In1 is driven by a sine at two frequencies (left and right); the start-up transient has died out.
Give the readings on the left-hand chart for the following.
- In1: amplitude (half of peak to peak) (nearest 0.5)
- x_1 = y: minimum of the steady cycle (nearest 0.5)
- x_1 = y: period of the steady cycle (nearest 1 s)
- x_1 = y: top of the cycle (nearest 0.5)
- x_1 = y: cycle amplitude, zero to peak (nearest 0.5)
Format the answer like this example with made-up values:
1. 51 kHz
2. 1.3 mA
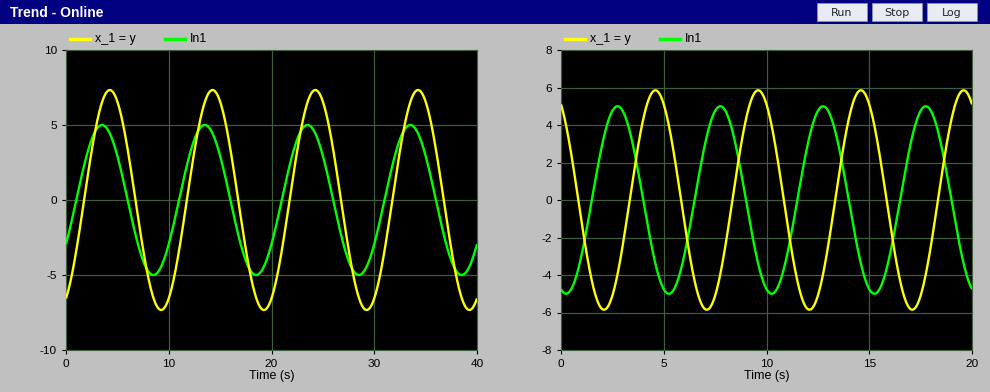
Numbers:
1. 5.0
2. -7.5
3. 10 s
4. 7.5
5. 7.5
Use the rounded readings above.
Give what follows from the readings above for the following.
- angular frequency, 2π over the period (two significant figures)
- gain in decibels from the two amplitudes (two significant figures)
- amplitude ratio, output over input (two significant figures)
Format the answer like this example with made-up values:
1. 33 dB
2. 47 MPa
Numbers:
1. 0.63 rad/s
2. 3.5 dB
3. 1.5
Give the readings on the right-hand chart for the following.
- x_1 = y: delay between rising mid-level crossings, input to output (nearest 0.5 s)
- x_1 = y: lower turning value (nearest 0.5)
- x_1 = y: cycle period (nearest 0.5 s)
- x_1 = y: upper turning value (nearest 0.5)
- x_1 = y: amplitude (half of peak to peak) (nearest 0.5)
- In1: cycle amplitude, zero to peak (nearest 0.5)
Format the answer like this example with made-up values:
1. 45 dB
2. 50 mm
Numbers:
1. 2.0 s
2. -6.0
3. 5.0 s
4. 6.0
5. 6.0
6. 5.0
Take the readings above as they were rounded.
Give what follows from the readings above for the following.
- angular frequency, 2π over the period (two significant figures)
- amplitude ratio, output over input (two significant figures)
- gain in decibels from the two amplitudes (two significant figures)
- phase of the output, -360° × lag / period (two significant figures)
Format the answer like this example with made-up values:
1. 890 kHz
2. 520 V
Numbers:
1. 1.3 rad/s
2. 1.2
3. 1.6 dB
4. -140°
